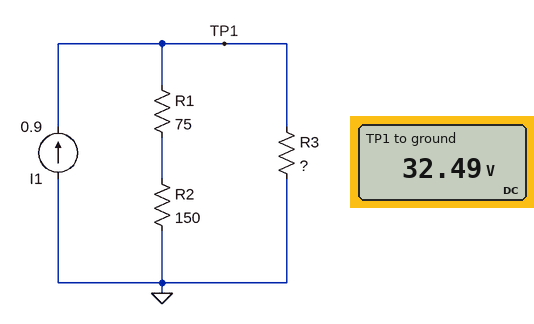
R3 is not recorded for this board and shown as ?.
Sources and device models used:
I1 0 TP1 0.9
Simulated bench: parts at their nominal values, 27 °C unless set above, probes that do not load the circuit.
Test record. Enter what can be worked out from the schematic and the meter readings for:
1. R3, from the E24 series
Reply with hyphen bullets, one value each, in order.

- 43 Ω
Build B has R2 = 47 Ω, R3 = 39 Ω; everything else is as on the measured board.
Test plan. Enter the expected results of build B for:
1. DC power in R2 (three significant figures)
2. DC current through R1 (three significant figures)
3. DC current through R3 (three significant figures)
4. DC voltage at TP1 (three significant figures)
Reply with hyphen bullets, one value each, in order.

- 2.23 W
- 218 mA
- 682 mA
- 26.6 V
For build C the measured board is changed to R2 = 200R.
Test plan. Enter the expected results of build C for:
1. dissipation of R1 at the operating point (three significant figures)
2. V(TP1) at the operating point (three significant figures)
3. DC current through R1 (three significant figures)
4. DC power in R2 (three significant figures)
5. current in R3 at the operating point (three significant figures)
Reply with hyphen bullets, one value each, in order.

- 1.11 W
- 33.5 V
- 122 mA
- 2.96 W
- 778 mA
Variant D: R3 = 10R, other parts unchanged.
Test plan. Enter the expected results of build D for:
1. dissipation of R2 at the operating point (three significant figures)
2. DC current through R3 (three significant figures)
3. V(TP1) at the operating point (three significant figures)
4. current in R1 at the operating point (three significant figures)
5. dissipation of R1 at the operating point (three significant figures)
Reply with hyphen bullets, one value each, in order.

- 220 mW
- 862 mA
- 8.62 V
- 38.3 mA
- 110 mW
